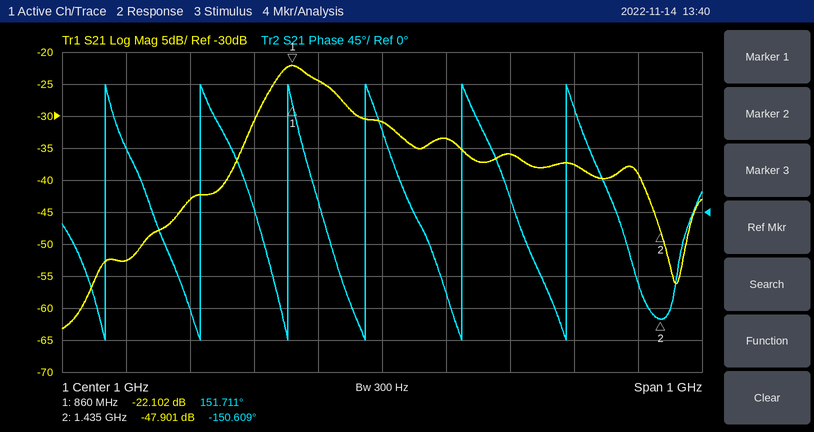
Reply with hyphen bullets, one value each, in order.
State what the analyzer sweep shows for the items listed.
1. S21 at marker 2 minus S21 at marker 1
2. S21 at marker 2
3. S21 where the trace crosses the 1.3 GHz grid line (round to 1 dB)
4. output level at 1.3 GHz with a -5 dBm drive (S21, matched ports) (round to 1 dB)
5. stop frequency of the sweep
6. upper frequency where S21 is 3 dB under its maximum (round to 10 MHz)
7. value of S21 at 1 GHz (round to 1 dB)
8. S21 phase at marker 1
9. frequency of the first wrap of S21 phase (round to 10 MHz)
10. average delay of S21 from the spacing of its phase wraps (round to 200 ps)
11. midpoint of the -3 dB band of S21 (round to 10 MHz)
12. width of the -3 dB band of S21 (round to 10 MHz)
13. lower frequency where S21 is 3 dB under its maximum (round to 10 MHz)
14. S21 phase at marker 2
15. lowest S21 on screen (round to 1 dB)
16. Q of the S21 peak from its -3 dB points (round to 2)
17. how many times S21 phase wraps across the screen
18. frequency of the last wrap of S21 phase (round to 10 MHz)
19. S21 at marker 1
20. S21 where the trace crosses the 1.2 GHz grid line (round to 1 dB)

- -25.799 dB
- -47.901 dB
- -38 dB
- -43 dBm
- 1.5 GHz
- 910 MHz
- -31 dB
- 151.711°
- 570 MHz
- 7.0 ns
- 870 MHz
- 80 MHz
- 830 MHz
- -150.609°
- -63 dB
- 10
- 6
- 1.29 GHz
- -22.102 dB
- -36 dB
